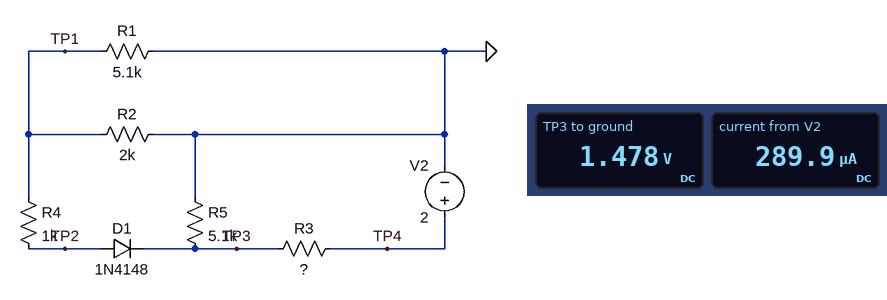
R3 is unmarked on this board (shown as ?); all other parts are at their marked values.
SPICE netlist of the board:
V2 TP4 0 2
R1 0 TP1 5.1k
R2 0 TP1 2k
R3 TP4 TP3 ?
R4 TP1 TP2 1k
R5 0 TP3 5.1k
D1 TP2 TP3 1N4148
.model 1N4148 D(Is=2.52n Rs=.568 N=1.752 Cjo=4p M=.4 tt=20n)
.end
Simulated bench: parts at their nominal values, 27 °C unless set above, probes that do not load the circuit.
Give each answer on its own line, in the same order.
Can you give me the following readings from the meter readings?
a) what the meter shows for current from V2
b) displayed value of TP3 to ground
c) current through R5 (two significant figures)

289.9 µA
1.478 V
290 µA
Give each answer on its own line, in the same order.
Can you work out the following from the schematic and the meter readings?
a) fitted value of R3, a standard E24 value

1.8 kΩ
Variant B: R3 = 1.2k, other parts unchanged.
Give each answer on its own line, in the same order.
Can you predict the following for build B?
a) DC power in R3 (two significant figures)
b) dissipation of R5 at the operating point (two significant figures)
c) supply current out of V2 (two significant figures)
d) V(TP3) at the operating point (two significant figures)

120 µW
510 µW
320 µA
1.6 V
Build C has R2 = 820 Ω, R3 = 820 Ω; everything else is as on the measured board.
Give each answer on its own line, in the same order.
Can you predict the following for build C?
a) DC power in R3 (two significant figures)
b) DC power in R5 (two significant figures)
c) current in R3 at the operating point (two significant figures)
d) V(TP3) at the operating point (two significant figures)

94 µW
580 µW
340 µA
1.7 V
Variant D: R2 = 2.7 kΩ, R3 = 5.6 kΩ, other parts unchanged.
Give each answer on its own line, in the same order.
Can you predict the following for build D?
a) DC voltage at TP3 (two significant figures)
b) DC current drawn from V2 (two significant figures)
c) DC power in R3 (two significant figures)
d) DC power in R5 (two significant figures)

950 mV
190 µA
200 µW
180 µW
